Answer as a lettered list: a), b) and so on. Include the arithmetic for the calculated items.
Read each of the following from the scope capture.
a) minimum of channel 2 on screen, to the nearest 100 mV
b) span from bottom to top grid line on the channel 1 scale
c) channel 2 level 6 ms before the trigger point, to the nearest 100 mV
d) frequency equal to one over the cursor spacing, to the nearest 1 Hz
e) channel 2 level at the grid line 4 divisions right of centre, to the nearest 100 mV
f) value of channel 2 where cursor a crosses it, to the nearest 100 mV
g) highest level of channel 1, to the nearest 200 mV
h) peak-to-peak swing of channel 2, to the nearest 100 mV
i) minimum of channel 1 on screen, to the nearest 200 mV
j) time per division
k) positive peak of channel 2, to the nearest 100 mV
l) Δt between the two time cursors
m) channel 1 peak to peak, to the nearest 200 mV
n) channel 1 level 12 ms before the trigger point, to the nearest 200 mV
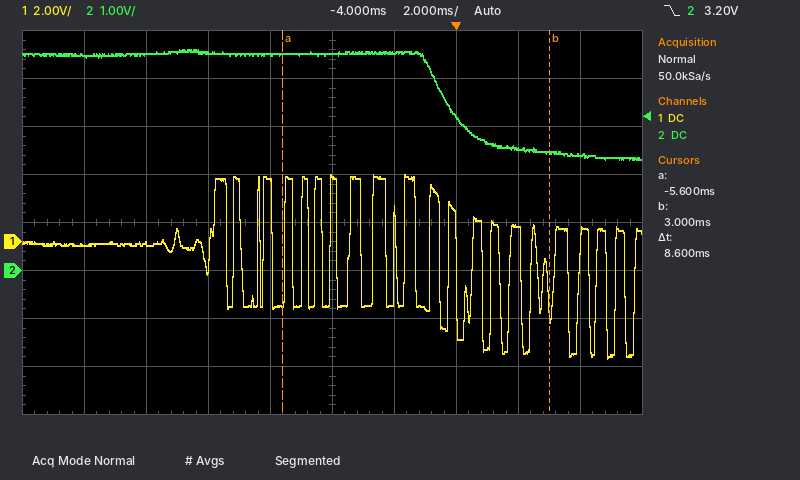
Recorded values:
a) 2.3 V
b) 16 V
c) 4.5 V
d) 1 / 8.6 ms ≈ 116 Hz
e) 2.4 V
f) 4.5 V
g) 2.8 V
h) 4.6 V − (2.3 V) = 2.3 V
i) -4.8 V
j) 2 ms
k) 4.6 V
l) 8.6 ms
m) 2.8 V − (-4.8 V) = 7.6 V
n) -200 mV
